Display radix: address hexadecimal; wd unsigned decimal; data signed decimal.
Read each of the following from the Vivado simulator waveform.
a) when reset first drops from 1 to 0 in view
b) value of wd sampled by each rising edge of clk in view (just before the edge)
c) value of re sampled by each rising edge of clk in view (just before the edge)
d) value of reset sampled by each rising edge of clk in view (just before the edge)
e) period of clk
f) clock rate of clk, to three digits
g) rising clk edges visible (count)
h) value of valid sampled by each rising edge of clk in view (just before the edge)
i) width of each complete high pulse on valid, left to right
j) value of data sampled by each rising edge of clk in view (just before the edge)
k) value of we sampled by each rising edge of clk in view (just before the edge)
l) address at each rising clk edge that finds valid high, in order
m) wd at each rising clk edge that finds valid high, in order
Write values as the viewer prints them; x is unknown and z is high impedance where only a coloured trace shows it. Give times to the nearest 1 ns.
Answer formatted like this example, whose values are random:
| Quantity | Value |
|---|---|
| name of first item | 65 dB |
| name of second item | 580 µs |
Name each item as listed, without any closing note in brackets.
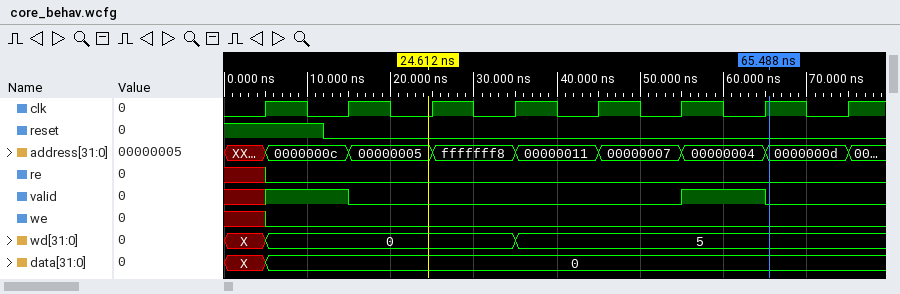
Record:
| Quantity | Value |
|---|---|
| when reset first drops from 1 to 0 in view | 12 ns |
| value of wd sampled by each rising edge of clk in view | X, 0, 0, 0, 5, 5, 5, 5 |
| value of re sampled by each rising edge of clk in view | x 0 0 0 0 0 0 0 |
| value of reset sampled by each rising edge of clk in view | 1 0 0 0 0 0 0 0 |
| period of clk | 10 ns |
| clock rate of clk, to three digits | 100 MHz |
| rising clk edges visible | 8 |
| value of valid sampled by each rising edge of clk in view | x 1 0 0 0 0 1 0 |
| width of each complete high pulse on valid, left to right | 10 ns |
| value of data sampled by each rising edge of clk in view | X, 0, 0, 0, 0, 0, 0, 0 |
| value of we sampled by each rising edge of clk in view | x 0 0 0 0 0 0 0 |
| address at each rising clk edge that finds valid high, in order | 0000000c, 00000004 |
| wd at each rising clk edge that finds valid high, in order | 0, 5 |
